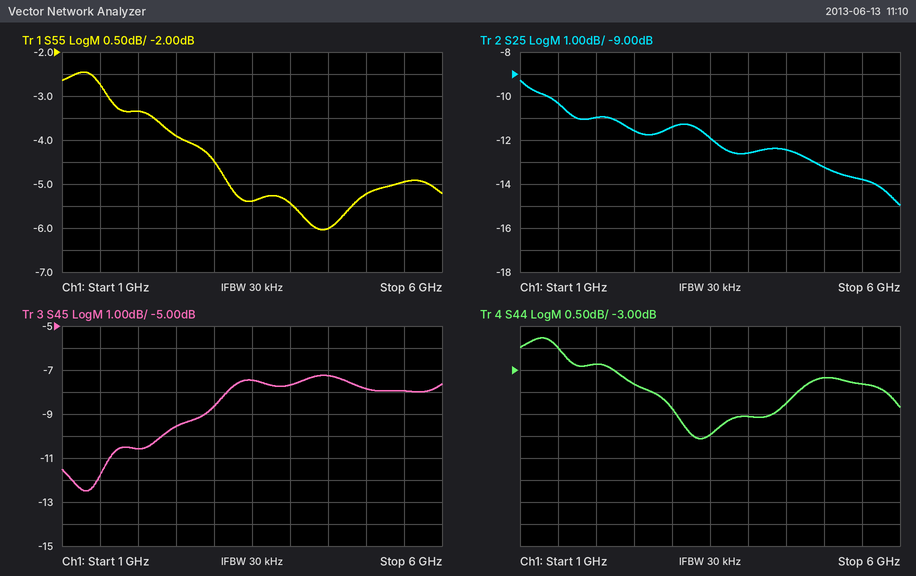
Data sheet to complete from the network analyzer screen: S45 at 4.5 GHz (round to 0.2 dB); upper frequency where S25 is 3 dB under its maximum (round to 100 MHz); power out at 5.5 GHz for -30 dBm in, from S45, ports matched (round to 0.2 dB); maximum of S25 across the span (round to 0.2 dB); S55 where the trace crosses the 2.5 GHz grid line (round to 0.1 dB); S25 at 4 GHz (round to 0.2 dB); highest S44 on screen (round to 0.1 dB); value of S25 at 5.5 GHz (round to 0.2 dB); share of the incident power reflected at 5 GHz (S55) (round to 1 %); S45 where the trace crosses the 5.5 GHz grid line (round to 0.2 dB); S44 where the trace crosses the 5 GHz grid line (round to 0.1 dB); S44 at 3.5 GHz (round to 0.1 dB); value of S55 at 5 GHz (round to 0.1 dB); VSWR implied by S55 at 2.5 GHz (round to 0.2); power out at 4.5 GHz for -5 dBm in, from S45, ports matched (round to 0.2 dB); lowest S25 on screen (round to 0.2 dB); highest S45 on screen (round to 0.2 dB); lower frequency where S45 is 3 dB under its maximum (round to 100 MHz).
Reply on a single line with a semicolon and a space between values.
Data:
-7.2 dB; 3.6 GHz; -38.0 dBm; -9.2 dB; -3.9 dB; -12.6 dB; -2.3 dB; -13.8 dB; 30 %; -8.0 dB; -3.2 dB; -4.5 dB; -5.2 dB; 4.6; -12.2 dBm; -15.0 dB; -7.2 dB; 2.2 GHz
